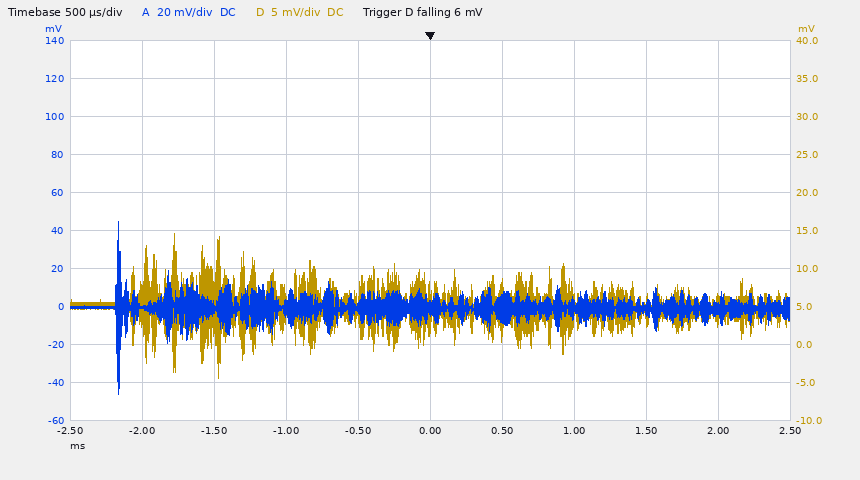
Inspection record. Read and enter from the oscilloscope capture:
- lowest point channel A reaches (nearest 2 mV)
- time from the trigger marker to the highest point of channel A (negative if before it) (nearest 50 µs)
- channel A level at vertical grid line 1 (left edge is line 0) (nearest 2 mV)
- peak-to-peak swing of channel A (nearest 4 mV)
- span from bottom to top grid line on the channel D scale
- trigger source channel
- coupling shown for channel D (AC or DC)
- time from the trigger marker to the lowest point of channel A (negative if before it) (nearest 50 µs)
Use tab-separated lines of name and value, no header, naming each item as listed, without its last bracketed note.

lowest point channel A reaches	-46 mV
time from the trigger marker to the highest point of channel A (negative if before it)	-2.15 ms
channel A level at vertical grid line 1 (left edge is line 0)	0 mV
peak-to-peak swing of channel A	92 mV
span from bottom to top grid line on the channel D scale	50 mV
trigger source channel	channel D
coupling shown for channel D	DC
time from the trigger marker to the lowest point of channel A (negative if before it)	-2.15 ms
